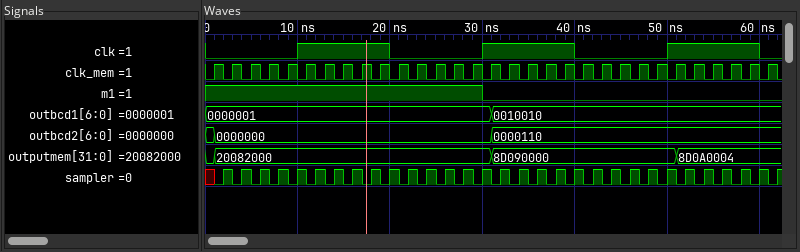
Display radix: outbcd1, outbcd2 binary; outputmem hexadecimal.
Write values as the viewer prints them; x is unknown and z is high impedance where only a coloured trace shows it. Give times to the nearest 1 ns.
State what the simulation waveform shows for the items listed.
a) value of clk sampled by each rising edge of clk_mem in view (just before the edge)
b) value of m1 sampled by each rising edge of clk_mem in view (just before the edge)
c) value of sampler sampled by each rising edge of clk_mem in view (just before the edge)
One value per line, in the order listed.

0 0 0 0 0 1 1 1 1 1 0 0 0 0 0 1 1 1 1 1 0 0 0 0 0 1 1 1 1 1 0
1 1 1 1 1 1 1 1 1 1 1 1 1 1 1 0 0 0 0 0 0 0 0 0 0 0 0 0 0 0 0
x 1 1 1 1 1 1 1 1 1 1 1 1 1 1 1 1 1 1 1 1 1 1 1 1 1 1 1 1 1 1
